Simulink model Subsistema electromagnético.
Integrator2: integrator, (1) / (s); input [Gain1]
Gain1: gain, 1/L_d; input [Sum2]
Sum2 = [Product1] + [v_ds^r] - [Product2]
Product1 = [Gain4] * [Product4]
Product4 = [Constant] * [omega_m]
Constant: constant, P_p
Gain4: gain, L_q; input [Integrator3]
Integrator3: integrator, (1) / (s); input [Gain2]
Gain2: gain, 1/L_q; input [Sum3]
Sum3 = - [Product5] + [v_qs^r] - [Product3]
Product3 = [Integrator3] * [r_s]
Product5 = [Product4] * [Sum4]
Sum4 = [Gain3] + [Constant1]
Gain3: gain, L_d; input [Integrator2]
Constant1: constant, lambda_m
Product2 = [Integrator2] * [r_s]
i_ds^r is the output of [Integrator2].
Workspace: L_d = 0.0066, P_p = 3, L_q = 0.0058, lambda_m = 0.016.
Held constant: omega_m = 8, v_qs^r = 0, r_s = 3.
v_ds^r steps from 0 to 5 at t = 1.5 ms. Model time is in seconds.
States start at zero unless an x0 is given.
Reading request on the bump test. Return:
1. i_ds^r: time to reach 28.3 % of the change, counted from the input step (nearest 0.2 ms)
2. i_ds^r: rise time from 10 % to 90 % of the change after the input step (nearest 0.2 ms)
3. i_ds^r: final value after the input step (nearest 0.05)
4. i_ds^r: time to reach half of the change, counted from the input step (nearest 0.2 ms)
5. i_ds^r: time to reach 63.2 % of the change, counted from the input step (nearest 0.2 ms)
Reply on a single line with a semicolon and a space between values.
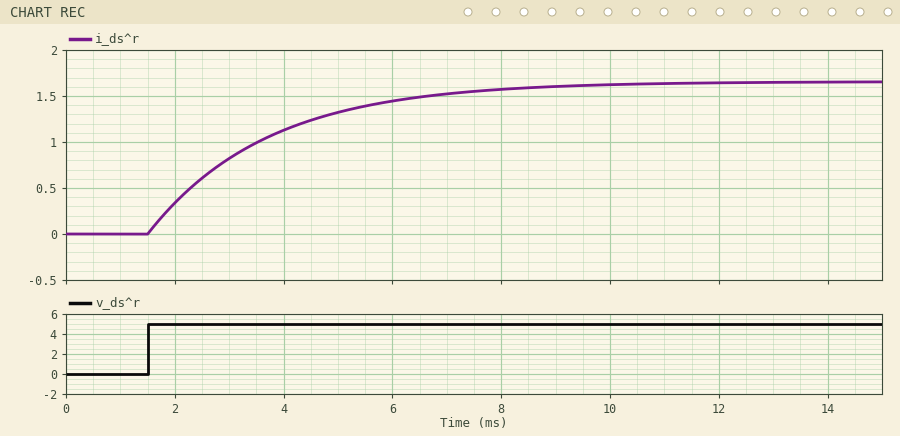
0.8 ms; 4.8 ms; 1.65; 1.6 ms; 2.2 ms
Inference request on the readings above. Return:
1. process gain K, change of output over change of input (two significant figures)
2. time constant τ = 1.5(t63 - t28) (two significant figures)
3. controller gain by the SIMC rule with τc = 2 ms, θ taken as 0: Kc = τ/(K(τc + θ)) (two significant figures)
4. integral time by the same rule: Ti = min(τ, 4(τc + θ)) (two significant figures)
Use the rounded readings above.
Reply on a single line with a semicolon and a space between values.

0.33; 2.1 ms; 3.2; 2.1 ms
